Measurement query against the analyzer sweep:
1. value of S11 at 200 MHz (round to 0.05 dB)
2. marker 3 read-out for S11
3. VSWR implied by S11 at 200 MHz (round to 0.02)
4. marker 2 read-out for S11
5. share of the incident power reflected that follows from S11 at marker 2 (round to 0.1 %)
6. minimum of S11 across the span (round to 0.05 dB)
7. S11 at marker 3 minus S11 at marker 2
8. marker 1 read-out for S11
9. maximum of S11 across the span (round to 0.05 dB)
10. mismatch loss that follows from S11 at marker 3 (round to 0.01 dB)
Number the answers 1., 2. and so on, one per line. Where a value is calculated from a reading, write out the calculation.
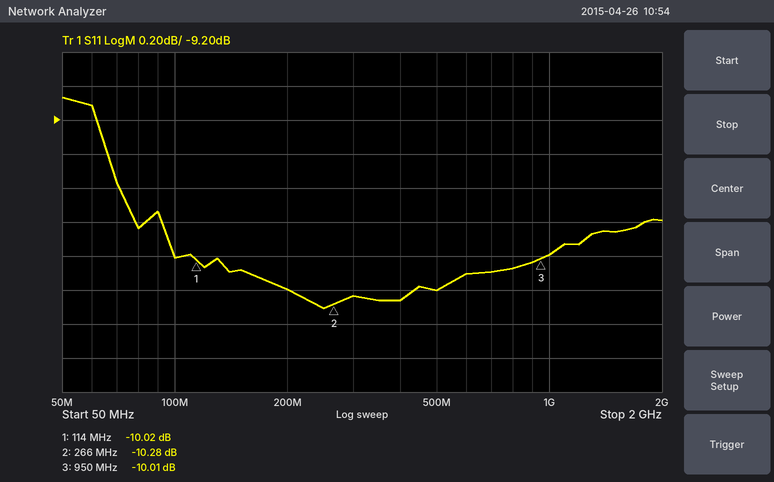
1. -10.20 dB
2. -10.01 dB
3. |Γ| = 10^(-10.2/20) = 0.3090; VSWR = (1 + 0.3090)/(1 − 0.3090) ≈ 1.89, so 1.90 to the nearest 0.02
4. -10.28 dB
5. 10^(-10.28/10) ≈ 9.4 %
6. -10.30 dB
7. -10.01 − (-10.28) = 0.27 dB
8. -10.02 dB
9. -9.05 dB
10. −10 log10(1 − 10^(-10.01/10)) ≈ 0.46 dB
